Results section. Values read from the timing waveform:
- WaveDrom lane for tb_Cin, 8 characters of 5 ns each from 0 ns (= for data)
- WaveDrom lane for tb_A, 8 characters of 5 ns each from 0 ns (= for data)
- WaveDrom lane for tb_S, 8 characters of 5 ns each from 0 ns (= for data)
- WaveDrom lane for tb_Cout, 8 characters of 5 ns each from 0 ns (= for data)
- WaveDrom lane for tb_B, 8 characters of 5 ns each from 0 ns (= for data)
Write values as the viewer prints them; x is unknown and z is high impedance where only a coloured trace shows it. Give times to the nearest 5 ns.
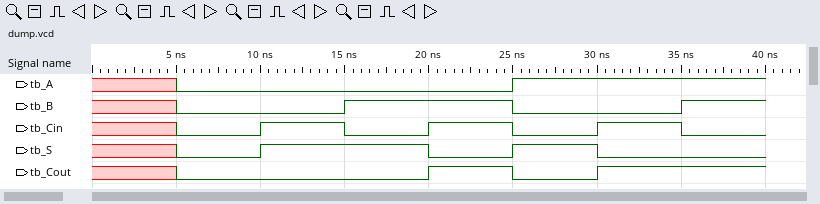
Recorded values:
{name: 'tb_Cin', wave: 'x0101010'}
{name: 'tb_A', wave: 'x0...1..'}
{name: 'tb_S', wave: 'x01.010.'}
{name: 'tb_Cout', wave: 'x0..101.'}
{name: 'tb_B', wave: 'x0.1.0.1'}
